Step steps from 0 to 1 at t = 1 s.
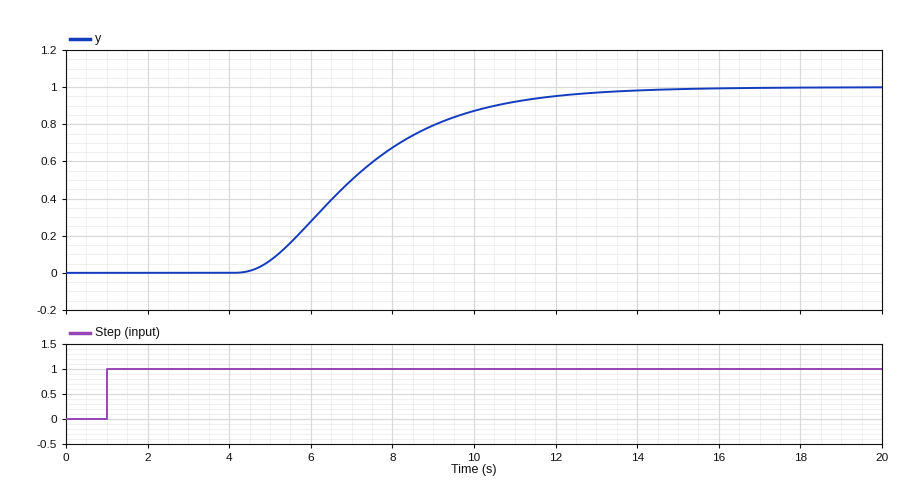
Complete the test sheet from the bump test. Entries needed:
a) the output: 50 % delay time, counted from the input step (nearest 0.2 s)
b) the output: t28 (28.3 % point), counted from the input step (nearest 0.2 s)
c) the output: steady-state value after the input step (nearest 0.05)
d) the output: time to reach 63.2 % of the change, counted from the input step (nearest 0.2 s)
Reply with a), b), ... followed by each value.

a) 6.0 s
b) 5.0 s
c) 1.00
d) 6.8 s
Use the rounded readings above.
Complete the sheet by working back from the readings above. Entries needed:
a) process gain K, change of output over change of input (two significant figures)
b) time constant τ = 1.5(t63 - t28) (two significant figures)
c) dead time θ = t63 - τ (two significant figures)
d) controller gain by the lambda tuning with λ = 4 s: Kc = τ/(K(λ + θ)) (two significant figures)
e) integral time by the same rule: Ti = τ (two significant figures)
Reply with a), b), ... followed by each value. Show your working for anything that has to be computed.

a) (1 - 0) / 1 = 1.0
b) 1.5 × (6.8 - 5) = 2.7 s
c) 6.8 - 2.7 = 4.1 s
d) 2.7 / (1 × (4 + 4.1)) = 0.33
e) 2.7 s
